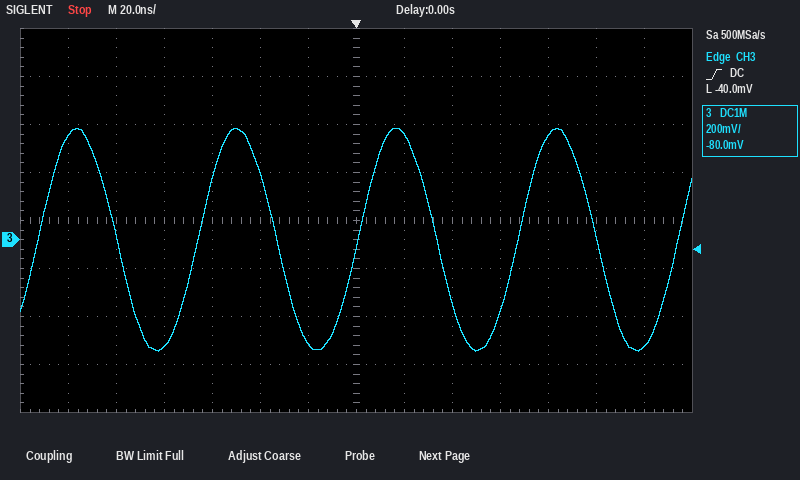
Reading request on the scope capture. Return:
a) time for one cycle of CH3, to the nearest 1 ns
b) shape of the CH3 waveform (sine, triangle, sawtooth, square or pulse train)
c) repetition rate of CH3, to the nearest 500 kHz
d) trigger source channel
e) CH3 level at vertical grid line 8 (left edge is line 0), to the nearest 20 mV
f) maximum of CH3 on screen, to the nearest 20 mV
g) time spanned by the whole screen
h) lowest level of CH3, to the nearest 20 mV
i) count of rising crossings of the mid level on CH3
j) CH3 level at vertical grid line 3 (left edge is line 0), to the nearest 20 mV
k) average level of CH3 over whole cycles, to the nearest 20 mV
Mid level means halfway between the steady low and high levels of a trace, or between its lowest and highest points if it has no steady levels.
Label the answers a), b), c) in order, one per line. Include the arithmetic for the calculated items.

a) 67 ns
b) sine
c) 1 / 67 ns ≈ 14.9 MHz, so 15.0 MHz to the nearest 500 kHz
d) CH3
e) 440 mV
f) 460 mV
g) 280 ns
h) -460 mV
i) 5
j) -440 mV
k) (460 mV + (-460 mV)) / 2 ≈ 0 mV
